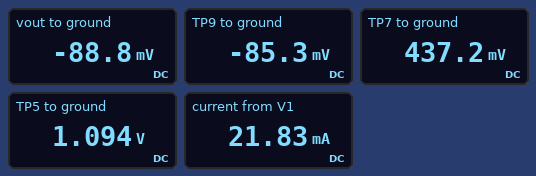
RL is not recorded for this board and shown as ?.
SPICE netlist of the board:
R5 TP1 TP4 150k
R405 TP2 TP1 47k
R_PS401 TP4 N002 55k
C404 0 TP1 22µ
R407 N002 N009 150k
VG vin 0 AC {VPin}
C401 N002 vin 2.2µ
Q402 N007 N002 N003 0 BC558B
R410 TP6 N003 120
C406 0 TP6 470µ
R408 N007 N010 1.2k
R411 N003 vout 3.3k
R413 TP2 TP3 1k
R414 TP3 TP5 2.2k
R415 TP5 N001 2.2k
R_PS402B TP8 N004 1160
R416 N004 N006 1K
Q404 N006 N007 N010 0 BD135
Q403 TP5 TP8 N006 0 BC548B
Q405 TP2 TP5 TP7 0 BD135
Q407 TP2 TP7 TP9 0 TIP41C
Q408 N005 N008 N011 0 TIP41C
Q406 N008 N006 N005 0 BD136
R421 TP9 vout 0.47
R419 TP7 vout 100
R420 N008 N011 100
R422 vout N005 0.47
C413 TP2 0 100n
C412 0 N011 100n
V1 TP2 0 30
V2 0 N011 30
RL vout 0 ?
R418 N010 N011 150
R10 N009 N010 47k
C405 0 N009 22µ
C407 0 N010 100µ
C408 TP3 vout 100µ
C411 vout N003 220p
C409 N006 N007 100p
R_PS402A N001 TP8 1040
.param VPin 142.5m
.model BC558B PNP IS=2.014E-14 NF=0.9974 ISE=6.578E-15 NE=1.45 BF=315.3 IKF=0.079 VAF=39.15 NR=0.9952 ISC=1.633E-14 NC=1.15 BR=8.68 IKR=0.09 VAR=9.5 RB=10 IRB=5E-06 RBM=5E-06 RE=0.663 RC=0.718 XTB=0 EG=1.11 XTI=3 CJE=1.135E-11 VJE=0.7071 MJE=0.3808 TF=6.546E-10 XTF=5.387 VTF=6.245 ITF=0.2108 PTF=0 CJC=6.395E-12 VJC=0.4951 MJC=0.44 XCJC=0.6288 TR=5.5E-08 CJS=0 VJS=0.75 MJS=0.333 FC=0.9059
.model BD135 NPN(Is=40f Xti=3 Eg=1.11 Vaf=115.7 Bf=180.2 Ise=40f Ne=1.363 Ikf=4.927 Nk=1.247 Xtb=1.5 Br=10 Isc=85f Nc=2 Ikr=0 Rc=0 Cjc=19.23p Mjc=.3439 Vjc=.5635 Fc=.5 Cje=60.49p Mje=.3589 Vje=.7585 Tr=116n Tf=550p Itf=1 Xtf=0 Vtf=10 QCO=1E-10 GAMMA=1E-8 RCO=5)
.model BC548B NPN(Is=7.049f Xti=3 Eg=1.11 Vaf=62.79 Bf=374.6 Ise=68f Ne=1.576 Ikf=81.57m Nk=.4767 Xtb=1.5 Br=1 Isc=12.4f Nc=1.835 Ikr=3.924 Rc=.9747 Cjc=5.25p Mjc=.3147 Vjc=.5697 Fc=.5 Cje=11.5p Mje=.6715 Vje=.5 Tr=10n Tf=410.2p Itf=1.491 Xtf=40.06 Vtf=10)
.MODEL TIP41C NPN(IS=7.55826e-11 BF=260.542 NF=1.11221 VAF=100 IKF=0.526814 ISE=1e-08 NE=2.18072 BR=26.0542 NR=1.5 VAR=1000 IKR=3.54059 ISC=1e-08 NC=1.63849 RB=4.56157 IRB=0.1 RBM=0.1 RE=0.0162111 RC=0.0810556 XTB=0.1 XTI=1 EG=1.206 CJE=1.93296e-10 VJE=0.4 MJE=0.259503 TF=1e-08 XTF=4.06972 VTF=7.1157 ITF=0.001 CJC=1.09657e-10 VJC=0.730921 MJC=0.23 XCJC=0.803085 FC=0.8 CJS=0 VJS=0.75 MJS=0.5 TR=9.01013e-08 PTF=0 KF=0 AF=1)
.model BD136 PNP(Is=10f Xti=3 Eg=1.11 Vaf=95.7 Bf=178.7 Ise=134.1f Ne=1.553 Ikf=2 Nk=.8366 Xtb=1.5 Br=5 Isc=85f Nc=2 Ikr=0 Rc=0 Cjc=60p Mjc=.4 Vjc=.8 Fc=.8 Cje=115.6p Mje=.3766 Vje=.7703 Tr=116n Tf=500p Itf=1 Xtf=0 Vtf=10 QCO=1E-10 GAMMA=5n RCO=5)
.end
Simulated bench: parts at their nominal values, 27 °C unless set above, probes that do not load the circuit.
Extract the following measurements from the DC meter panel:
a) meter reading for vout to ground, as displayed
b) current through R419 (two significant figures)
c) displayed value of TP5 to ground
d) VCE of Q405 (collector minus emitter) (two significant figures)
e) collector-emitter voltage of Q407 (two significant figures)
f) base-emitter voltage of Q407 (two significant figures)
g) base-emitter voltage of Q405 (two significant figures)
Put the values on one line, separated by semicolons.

-88.8 mV; 5.3 mA; 1.094 V; 30 V; 30 V; 520 mV; 660 mV
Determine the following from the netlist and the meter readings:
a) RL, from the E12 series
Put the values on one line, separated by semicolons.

3.3 Ω
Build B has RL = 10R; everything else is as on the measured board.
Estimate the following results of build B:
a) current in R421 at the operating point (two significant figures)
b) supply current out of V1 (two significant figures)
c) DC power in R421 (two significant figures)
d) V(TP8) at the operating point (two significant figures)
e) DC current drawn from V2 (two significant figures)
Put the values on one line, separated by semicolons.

9.5 mA; 24 mA; 42 µW; -72 mV; 33 mA
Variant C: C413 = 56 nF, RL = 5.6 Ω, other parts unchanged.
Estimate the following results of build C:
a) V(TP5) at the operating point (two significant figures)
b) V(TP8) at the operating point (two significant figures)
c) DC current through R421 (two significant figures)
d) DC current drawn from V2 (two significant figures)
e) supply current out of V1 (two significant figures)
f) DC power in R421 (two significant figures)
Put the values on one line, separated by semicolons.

1.1 V; -75 mV; 8.6 mA; 39 mA; 23 mA; 35 µW
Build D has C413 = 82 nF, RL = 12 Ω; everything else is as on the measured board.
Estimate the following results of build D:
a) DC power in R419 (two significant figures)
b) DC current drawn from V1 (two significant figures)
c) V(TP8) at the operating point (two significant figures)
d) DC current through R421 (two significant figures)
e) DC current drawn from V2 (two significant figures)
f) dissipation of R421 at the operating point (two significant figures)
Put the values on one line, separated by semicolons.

2.9 mW; 24 mA; -71 mV; 9.7 mA; 32 mA; 44 µW
